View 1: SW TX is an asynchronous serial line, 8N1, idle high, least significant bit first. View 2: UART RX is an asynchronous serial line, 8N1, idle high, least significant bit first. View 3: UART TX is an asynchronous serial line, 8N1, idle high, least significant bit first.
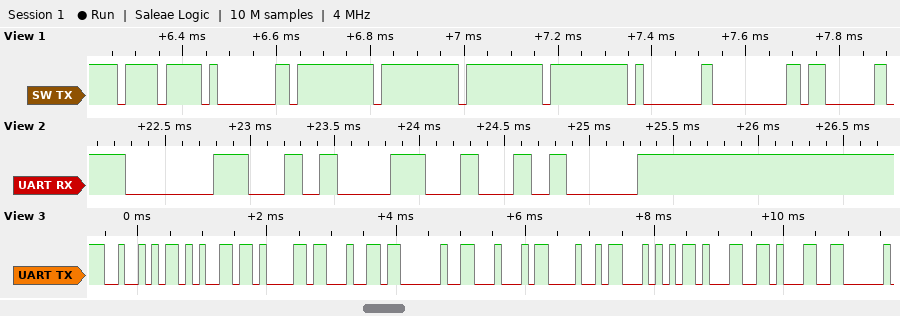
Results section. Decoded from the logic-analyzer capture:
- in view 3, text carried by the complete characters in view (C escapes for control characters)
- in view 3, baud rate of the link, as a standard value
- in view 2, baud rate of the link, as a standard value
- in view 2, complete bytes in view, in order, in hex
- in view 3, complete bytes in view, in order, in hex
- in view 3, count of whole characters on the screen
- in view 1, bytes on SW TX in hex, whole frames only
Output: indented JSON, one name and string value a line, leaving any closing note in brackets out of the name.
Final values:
{
  "in view 3, text carried by the complete characters in view": "\"Read DHT11\"",
  "in view 3, baud rate of the link, as a standard value": "9600 baud",
  "in view 2, baud rate of the link, as a standard value": "9600 baud",
  "in view 2, complete bytes in view, in order, in hex": "30 31 0A",
  "in view 3, complete bytes in view, in order, in hex": "52 65 61 64 20 44 48 54 31 31",
  "in view 3, count of whole characters on the screen": "10",
  "in view 1, bytes on SW TX in hex, whole frames only": "EF 01 FF FF FF FF 01 00 03"
}
